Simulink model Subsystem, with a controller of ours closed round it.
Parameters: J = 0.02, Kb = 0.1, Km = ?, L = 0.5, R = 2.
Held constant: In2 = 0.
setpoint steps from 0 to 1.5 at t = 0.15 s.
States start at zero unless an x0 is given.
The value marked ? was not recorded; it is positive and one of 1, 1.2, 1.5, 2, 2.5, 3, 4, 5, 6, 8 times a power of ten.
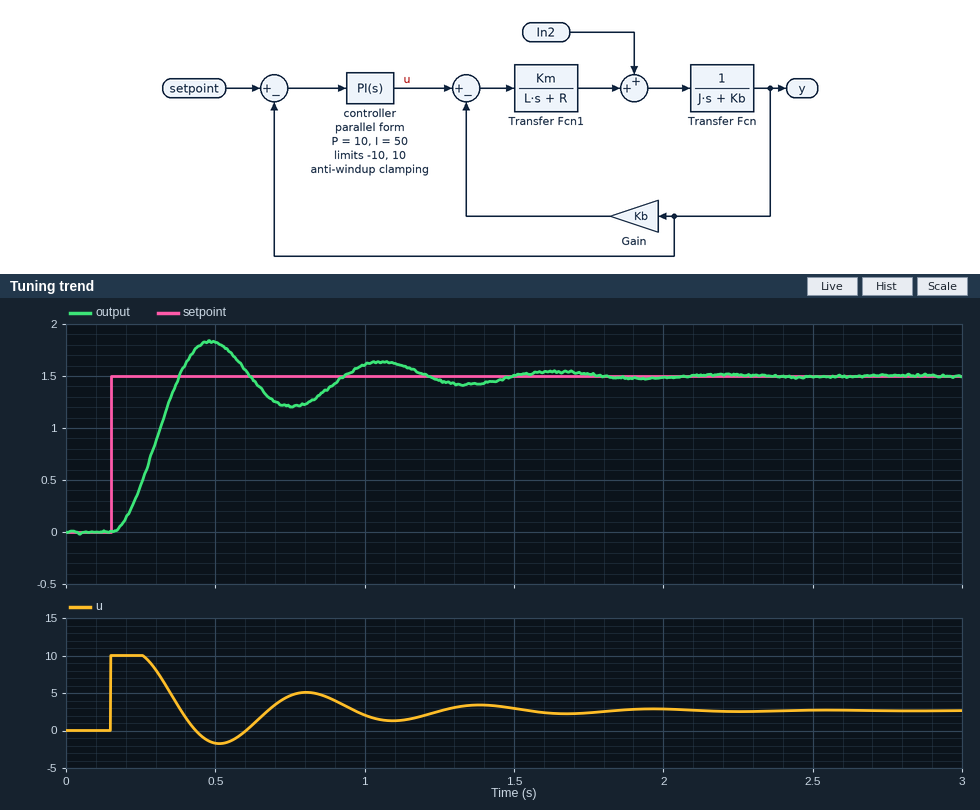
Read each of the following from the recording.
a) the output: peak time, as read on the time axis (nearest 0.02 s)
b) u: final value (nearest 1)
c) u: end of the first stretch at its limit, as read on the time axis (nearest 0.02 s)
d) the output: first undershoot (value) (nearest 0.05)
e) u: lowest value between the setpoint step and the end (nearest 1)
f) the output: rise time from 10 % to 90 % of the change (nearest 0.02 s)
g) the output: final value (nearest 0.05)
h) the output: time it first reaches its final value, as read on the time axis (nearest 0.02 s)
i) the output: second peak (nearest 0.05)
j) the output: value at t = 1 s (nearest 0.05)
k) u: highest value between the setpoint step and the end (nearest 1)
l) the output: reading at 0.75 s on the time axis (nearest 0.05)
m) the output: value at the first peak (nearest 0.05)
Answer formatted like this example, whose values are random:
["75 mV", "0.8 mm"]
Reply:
["0.48 s", "3", "0.26 s", "1.20", "-2", "0.16 s", "1.50", "0.38 s", "1.65", "1.60", "10", "1.20", "1.85"]
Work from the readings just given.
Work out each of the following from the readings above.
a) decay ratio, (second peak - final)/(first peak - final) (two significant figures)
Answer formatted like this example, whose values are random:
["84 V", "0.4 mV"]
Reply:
["0.43"]
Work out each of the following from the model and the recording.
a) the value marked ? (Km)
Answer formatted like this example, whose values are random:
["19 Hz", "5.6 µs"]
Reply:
["0.12"]
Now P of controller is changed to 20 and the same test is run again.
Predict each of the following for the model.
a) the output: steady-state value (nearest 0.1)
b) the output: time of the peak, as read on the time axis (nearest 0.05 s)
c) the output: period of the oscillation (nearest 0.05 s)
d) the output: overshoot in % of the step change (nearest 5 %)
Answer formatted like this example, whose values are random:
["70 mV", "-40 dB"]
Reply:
["1.5", "0.45 s", "0.40 s", "15 %"]
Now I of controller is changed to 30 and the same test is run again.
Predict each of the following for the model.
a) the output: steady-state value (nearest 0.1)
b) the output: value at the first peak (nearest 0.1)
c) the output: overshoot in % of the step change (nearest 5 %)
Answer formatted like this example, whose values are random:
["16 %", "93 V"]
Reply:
["1.5", "1.7", "15 %"]
